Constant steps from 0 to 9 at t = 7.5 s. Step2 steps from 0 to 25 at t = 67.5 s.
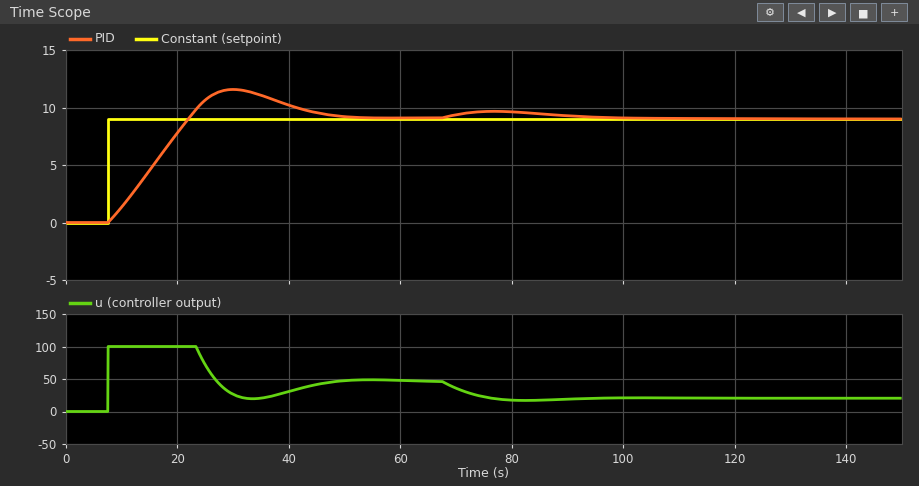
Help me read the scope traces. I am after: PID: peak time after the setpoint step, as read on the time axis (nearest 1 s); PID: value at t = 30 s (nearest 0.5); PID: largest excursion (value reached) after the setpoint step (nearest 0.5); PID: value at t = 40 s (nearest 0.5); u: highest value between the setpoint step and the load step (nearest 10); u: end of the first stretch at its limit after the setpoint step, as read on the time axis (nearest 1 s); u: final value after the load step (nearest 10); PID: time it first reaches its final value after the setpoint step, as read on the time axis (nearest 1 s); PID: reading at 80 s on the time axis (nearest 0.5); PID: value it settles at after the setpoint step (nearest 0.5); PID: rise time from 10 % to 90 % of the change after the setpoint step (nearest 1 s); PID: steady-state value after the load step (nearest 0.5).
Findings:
30 s
11.5
11.5
10.0
100
23 s
20
22 s
9.5
9.0
11 s
9.0
